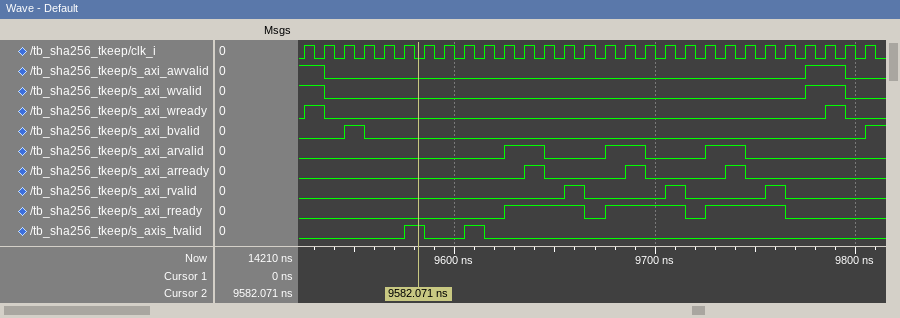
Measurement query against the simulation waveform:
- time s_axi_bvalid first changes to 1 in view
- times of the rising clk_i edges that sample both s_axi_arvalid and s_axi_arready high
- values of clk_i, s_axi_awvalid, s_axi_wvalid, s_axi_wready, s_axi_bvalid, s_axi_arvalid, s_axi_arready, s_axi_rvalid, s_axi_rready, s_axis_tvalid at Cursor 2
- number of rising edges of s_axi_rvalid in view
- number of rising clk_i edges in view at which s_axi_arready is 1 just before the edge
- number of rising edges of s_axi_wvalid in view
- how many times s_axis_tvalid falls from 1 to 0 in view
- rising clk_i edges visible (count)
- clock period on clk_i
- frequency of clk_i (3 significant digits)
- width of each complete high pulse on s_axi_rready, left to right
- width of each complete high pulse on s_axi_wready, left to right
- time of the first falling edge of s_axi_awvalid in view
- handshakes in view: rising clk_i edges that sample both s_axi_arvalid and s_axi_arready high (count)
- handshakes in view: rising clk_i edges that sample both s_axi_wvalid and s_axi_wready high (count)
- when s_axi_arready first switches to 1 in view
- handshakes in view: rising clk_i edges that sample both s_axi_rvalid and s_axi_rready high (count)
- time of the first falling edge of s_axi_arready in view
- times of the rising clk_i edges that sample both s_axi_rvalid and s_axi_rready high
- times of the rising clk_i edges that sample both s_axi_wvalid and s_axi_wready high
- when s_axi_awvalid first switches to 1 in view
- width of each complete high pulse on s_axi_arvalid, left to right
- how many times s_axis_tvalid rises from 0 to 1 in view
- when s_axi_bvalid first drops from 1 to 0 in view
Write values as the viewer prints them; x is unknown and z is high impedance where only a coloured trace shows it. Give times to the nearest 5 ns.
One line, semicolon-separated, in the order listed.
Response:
9545 ns; 9645 ns, 9695 ns, 9745 ns; clk_i=0, s_axi_awvalid=0, s_axi_wvalid=0, s_axi_wready=0, s_axi_bvalid=0, s_axi_arvalid=0, s_axi_arready=0, s_axi_rvalid=0, s_axi_rready=0, s_axis_tvalid=1; 3; 3; 1; 2; 29; 10 ns; 100 MHz; 40 ns, 40 ns, 40 ns; 10 ns, 10 ns; 9535 ns; 3; 2; 9635 ns; 3; 9645 ns; 9665 ns, 9715 ns, 9765 ns; 9535 ns, 9795 ns; 9775 ns; 20 ns, 20 ns, 20 ns; 2; 9555 ns
